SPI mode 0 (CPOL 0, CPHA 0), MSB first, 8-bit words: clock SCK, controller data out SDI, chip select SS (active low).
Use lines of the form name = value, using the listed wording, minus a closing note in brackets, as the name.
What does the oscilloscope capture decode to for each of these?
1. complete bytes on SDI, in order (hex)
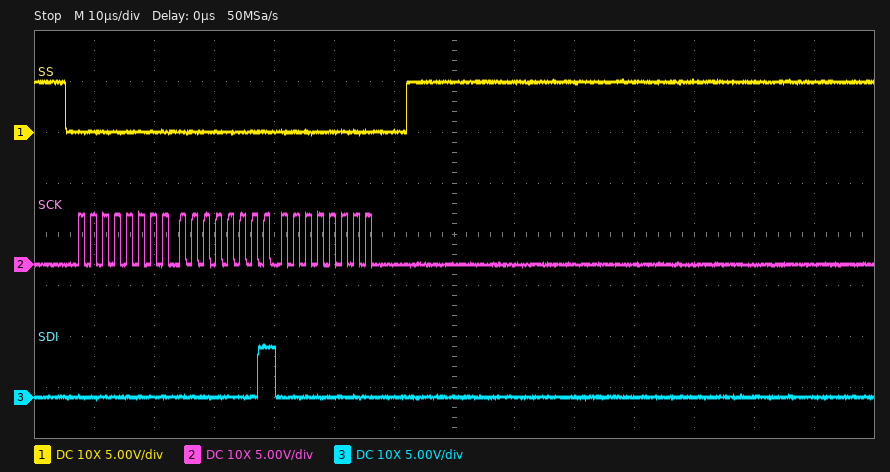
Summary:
complete bytes on SDI, in order = 0x00 0x01 0x00
